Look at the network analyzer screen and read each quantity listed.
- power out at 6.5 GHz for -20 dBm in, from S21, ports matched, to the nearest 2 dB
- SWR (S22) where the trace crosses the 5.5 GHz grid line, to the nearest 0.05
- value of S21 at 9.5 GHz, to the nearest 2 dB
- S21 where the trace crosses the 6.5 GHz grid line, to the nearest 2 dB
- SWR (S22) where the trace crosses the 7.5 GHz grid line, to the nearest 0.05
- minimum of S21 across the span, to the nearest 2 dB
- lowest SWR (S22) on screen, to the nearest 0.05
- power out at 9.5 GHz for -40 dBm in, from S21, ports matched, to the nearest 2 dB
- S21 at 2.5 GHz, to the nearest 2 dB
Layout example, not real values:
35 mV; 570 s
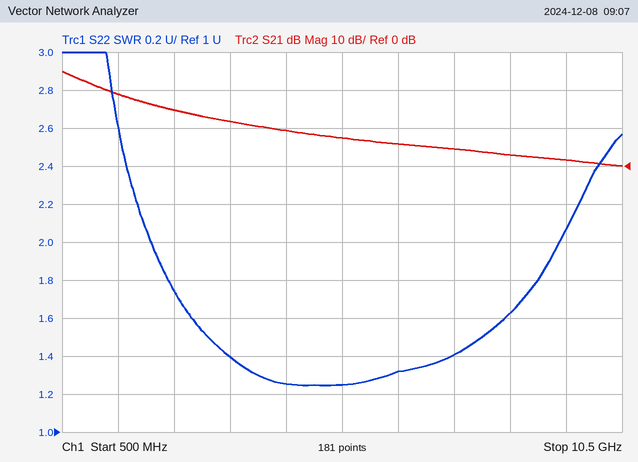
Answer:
-14 dBm; 1.25; 2 dB; 6 dB; 1.40; 0 dB; 1.25; -38 dBm; 14 dB
